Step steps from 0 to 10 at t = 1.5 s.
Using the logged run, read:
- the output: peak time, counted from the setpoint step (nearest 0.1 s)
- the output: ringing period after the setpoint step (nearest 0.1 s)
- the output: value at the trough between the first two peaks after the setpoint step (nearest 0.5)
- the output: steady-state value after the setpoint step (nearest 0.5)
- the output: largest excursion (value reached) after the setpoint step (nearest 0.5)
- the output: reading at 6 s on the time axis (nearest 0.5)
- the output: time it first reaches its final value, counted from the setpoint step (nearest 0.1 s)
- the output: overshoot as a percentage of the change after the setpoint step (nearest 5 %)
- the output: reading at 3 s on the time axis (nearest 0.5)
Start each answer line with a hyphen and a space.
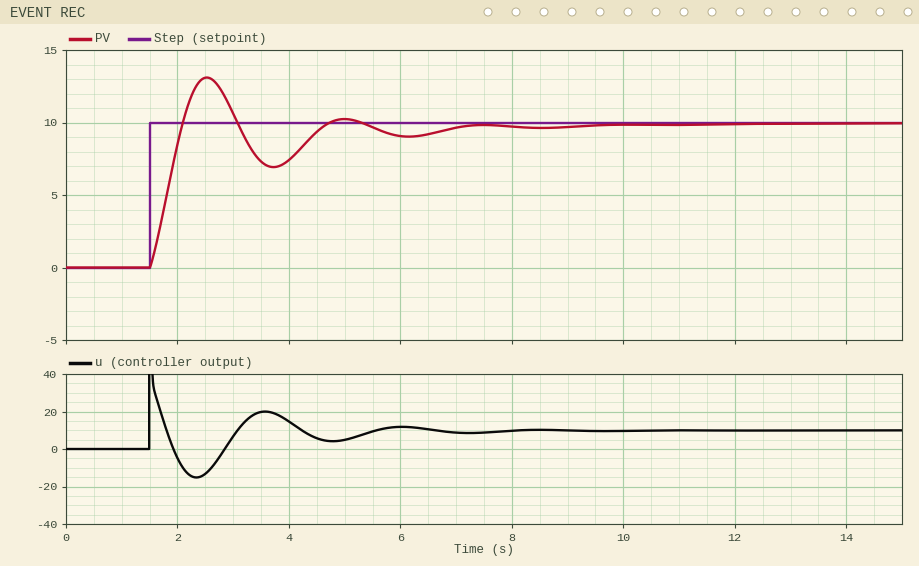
- 1.0 s
- 2.5 s
- 7.0
- 10.0
- 13.0
- 9.0
- 0.6 s
- 30 %
- 10.5
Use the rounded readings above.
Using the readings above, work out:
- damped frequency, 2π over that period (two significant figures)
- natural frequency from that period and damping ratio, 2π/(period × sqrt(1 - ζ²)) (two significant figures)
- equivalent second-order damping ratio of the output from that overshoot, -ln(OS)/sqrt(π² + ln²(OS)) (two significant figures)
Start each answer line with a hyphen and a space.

- 2.5 rad/s
- 2.7 rad/s
- 0.36
